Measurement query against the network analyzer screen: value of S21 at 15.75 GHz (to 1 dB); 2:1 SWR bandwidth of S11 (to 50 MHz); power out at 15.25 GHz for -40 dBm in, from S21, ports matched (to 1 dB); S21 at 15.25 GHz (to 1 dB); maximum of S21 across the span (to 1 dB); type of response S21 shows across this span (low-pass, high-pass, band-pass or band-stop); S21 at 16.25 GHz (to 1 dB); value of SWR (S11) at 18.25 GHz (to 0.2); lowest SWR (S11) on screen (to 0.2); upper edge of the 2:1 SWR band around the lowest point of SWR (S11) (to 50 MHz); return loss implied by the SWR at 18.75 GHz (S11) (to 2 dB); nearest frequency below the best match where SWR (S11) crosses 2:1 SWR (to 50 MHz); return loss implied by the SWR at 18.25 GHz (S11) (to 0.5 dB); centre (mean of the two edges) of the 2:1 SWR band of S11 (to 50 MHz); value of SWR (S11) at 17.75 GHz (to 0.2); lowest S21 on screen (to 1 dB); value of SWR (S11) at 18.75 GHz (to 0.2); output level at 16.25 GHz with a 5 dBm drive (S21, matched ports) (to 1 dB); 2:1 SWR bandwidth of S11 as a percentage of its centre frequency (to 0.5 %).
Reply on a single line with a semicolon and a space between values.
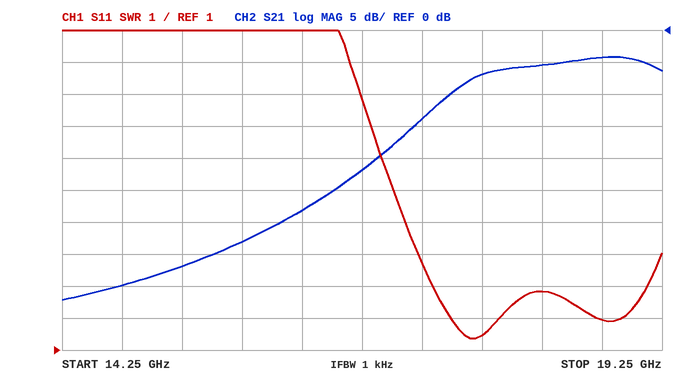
-33 dB; 400 MHz; -77 dBm; -37 dB; -4 dB; high-pass; -28 dB; 2.8; 1.4; 17.90 GHz; 10 dB; 17.50 GHz; 6.5 dB; 17.70 GHz; 1.4; -42 dB; 2.0; -23 dBm; 2.5 %
